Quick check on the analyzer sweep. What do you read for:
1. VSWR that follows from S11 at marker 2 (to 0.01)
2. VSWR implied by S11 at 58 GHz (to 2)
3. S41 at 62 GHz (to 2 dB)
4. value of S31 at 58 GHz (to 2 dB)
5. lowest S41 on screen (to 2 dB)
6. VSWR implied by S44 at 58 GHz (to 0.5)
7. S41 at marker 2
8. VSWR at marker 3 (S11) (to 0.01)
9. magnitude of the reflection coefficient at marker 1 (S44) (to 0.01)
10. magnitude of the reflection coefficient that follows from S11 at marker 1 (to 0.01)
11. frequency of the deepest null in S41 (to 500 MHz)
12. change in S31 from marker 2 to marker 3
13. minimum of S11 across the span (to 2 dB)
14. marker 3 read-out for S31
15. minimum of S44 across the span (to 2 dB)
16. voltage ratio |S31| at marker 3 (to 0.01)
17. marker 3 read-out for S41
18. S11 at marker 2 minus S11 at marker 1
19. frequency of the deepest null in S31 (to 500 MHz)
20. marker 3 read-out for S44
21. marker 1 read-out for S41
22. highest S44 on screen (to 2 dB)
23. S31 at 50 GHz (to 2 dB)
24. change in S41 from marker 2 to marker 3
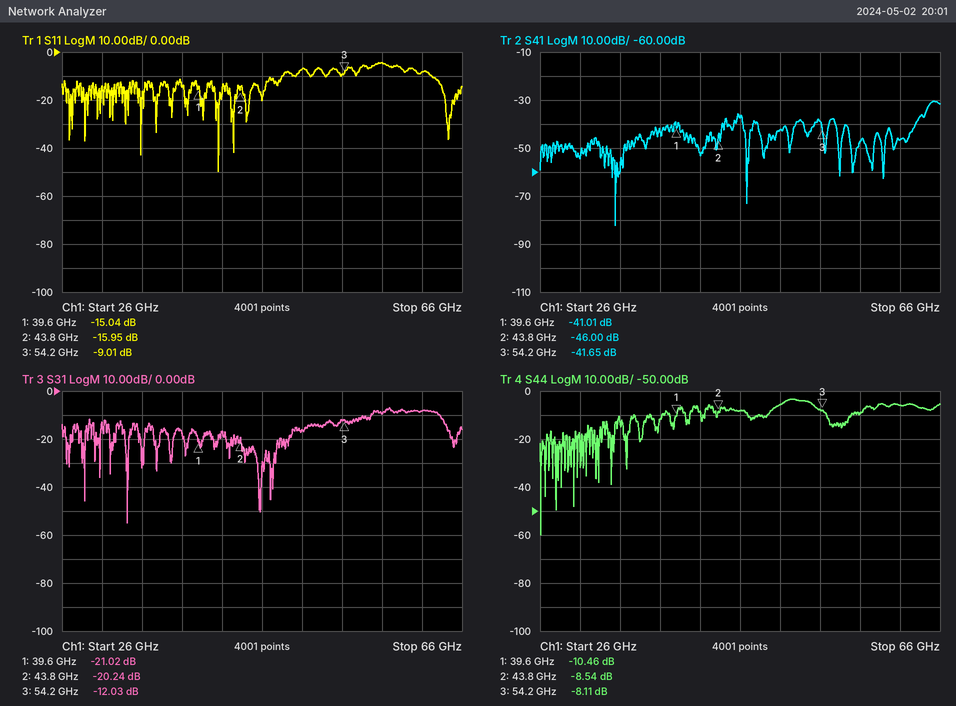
1.38
4
-46 dB
-10 dB
-82 dB
2.0
-46.00 dB
2.10
0.30
0.18
33.5 GHz
8.21 dB
-50 dB
-12.03 dB
-60 dB
0.25
-41.65 dB
-0.91 dB
32.5 GHz
-8.11 dB
-41.01 dB
-4 dB
-16 dB
4.35 dB
